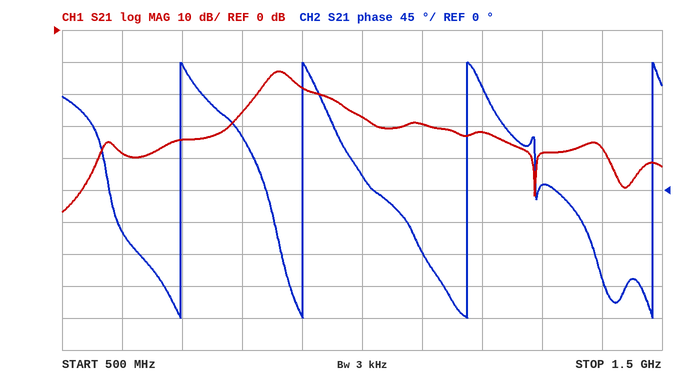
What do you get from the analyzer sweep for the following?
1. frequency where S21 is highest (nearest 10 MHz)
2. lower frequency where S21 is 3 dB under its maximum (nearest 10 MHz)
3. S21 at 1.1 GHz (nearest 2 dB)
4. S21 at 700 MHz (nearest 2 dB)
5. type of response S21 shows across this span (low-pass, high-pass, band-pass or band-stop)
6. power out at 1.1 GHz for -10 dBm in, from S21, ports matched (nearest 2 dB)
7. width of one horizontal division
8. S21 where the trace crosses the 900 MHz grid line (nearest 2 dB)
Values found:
860 MHz
840 MHz
-30 dB
-34 dB
band-pass
-40 dBm
100 MHz
-18 dB
